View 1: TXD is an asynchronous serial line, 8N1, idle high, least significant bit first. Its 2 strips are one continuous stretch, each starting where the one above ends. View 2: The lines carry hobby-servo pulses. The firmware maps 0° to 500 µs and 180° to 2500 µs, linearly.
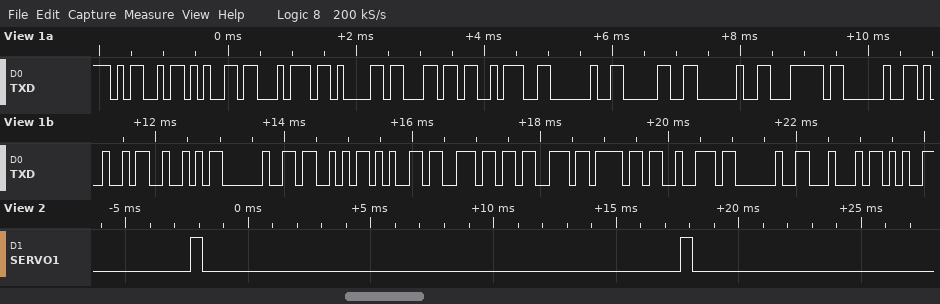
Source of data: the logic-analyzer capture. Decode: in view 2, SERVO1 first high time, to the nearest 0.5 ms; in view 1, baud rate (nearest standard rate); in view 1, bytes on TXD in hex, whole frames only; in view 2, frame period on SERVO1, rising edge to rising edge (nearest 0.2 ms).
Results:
0.5 ms
9600 baud
4D 65 74 61 6C 3A 20 30 20 7C 20 49 52 20 53 65 6E 73 6F 72 20 44
20.0 ms
